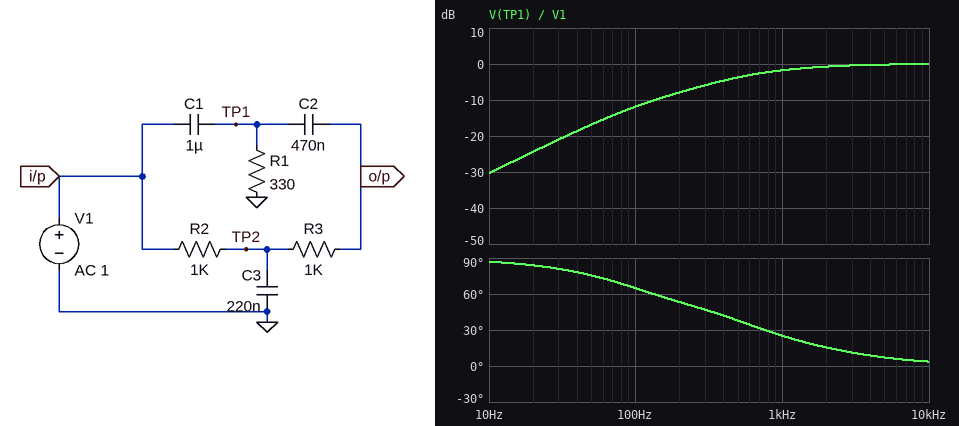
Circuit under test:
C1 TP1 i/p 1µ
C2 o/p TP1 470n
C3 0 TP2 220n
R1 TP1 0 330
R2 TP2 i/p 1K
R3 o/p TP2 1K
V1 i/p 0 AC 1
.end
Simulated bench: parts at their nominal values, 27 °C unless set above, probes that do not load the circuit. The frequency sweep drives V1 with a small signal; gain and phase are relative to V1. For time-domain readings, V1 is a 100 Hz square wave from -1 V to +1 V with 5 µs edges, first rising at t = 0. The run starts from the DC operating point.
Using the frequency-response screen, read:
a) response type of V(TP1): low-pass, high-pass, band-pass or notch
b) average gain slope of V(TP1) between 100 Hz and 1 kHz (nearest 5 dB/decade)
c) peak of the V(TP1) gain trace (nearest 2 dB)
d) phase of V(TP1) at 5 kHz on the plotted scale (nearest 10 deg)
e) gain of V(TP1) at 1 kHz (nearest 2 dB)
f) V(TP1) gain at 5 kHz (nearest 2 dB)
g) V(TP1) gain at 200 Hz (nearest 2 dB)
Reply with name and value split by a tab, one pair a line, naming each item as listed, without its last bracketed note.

response type of V(TP1): low-pass, high-pass, band-pass or notch	high-pass
average gain slope of V(TP1) between 100 Hz and 1 kHz	10 dB/decade
peak of the V(TP1) gain trace	0 dB
phase of V(TP1) at 5 kHz on the plotted scale	10 deg
gain of V(TP1) at 1 kHz	-2 dB
V(TP1) gain at 5 kHz	0 dB
V(TP1) gain at 200 Hz	-8 dB
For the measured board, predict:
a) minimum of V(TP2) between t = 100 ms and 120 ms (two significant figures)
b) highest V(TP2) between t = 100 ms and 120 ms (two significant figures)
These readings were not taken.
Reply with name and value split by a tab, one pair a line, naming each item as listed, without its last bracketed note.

minimum of V(TP2) between t = 100 ms and 120 ms	-980 mV
highest V(TP2) between t = 100 ms and 120 ms	980 mV
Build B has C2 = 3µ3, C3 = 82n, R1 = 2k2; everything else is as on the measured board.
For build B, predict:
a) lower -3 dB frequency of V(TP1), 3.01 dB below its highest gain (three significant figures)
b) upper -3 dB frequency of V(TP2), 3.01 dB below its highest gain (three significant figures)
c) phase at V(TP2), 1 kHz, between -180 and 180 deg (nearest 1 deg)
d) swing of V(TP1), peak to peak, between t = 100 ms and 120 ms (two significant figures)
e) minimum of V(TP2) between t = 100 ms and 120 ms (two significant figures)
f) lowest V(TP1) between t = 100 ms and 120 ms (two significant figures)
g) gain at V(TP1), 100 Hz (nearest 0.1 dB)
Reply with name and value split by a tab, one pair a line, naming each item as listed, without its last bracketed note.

lower -3 dB frequency of V(TP1), 3.01 dB below its highest gain	85.5 Hz
upper -3 dB frequency of V(TP2), 3.01 dB below its highest gain	3.77 kHz
phase at V(TP2), 1 kHz, between -180 and 180 deg	-12 deg
swing of V(TP1), peak to peak, between t = 100 ms and 120 ms	3.0 V
minimum of V(TP2) between t = 100 ms and 120 ms	-1.1 V
lowest V(TP1) between t = 100 ms and 120 ms	-1.5 V
gain at V(TP1), 100 Hz	-2.7 dB
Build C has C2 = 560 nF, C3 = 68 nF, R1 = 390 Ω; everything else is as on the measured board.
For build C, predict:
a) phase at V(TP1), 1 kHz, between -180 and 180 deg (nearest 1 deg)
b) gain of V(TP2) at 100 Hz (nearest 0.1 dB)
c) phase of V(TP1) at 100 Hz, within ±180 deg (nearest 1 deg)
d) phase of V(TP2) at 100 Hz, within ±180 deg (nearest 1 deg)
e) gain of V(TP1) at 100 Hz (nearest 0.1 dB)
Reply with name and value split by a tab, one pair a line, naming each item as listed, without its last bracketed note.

phase at V(TP1), 1 kHz, between -180 and 180 deg	21 deg
gain of V(TP2) at 100 Hz	-1.9 dB
phase of V(TP1) at 100 Hz, within ±180 deg	61 deg
phase of V(TP2) at 100 Hz, within ±180 deg	-13 deg
gain of V(TP1) at 100 Hz	-10.3 dB
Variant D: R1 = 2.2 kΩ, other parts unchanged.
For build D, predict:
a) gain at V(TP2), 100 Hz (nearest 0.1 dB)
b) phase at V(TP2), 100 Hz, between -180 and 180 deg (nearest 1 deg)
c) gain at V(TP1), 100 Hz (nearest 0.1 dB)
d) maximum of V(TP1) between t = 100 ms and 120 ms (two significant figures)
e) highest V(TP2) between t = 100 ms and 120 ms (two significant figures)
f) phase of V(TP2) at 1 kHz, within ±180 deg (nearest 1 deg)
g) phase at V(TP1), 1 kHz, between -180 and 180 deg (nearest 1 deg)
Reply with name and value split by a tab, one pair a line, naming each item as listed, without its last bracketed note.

gain at V(TP2), 100 Hz	-1.3 dB
phase at V(TP2), 100 Hz, between -180 and 180 deg	-7 deg
gain at V(TP1), 100 Hz	-1.7 dB
maximum of V(TP1) between t = 100 ms and 120 ms	1.6 V
highest V(TP2) between t = 100 ms and 120 ms	930 mV
phase of V(TP2) at 1 kHz, within ±180 deg	-30 deg
phase at V(TP1), 1 kHz, between -180 and 180 deg	5 deg
